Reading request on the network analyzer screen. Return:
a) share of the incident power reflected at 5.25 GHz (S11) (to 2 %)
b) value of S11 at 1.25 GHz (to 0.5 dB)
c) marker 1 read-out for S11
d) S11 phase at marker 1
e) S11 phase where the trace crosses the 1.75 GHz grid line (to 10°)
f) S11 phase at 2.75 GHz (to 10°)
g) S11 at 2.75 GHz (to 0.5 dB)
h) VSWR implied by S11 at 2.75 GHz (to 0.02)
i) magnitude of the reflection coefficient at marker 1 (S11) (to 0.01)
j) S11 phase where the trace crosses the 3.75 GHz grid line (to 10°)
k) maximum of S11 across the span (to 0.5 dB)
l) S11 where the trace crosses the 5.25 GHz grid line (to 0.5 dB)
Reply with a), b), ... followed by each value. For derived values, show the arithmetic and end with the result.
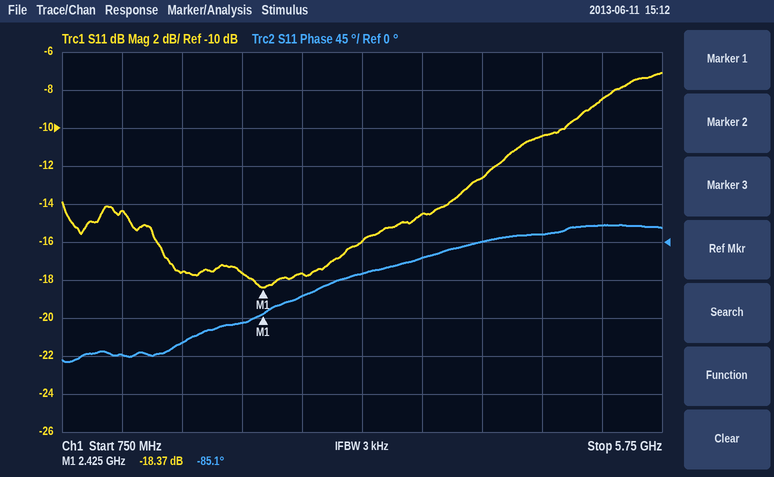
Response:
a) 10^(-8.5/10) ≈ 14 %
b) -14.5 dB
c) -18.37 dB
d) -85.1°
e) -120°
f) -60°
g) -17.5 dB
h) |Γ| = 10^(-17.5/20) = 0.1334; VSWR = (1 + 0.1334)/(1 − 0.1334) ≈ 1.31, so 1.30 to the nearest 0.02
i) 10^(-18.37/20) ≈ 0.12
j) -20°
k) -7.0 dB
l) -8.5 dB
